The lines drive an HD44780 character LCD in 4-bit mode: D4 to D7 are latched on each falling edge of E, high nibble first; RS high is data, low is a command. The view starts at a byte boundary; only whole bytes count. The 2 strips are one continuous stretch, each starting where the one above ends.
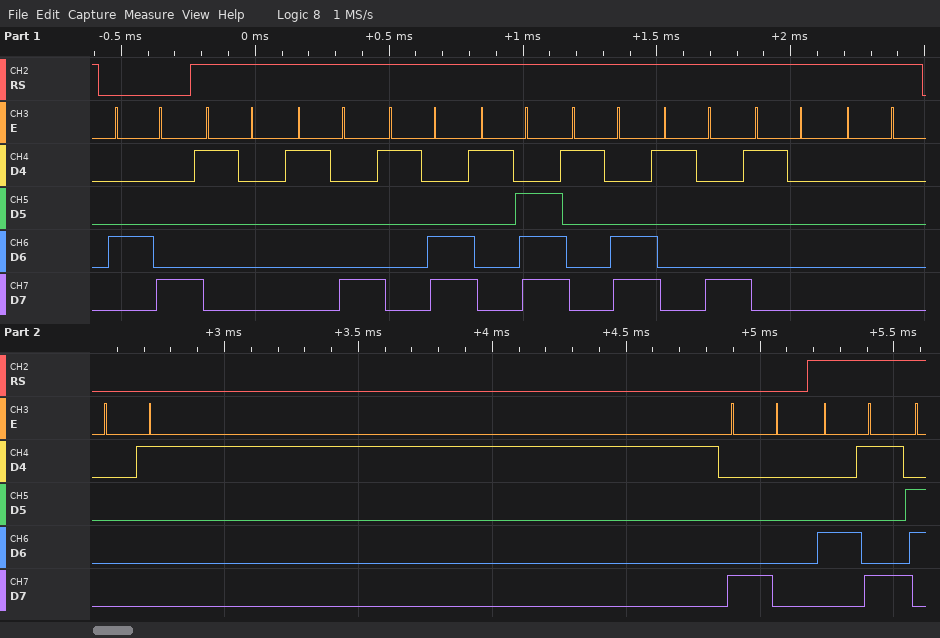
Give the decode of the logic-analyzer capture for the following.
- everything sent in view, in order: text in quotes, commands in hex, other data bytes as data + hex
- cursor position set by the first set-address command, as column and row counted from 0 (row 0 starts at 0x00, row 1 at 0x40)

0x48 data 10 18 1C 1E 1C 18 10 00 0x01 0x80 "I"
column 0, row 0
